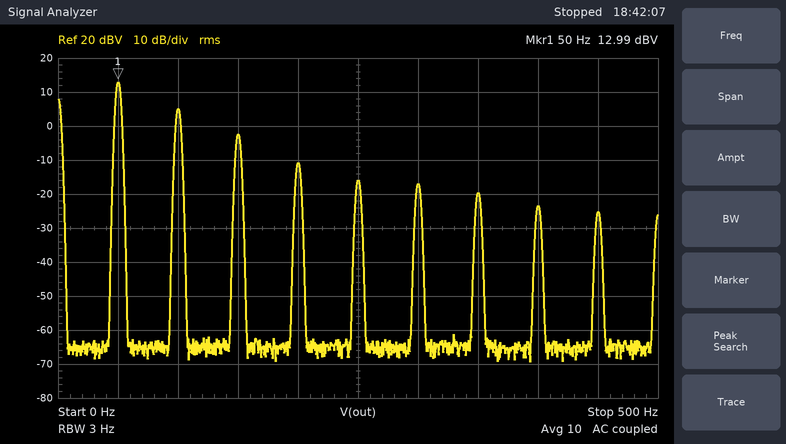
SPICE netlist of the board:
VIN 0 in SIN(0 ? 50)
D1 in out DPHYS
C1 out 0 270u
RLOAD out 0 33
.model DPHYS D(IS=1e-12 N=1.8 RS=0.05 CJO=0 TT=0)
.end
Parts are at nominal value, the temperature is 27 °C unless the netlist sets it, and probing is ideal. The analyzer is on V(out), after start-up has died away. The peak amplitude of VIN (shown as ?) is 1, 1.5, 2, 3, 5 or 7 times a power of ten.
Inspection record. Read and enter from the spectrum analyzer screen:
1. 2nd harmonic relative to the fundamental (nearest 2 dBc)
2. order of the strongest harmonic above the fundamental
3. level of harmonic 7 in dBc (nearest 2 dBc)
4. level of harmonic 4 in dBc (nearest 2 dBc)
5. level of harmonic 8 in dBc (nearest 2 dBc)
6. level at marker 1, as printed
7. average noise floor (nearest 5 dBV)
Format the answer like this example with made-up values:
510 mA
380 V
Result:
-8 dBc
2
-32 dBc
-24 dBc
-36 dBc
12.99 dBV
-65 dBV
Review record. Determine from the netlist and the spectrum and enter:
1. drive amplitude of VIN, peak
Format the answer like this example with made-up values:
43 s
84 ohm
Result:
20 V
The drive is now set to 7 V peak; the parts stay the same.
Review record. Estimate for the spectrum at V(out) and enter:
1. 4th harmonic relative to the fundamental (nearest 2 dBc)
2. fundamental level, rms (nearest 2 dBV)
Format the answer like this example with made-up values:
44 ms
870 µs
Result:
-22 dBc
2 dBV
